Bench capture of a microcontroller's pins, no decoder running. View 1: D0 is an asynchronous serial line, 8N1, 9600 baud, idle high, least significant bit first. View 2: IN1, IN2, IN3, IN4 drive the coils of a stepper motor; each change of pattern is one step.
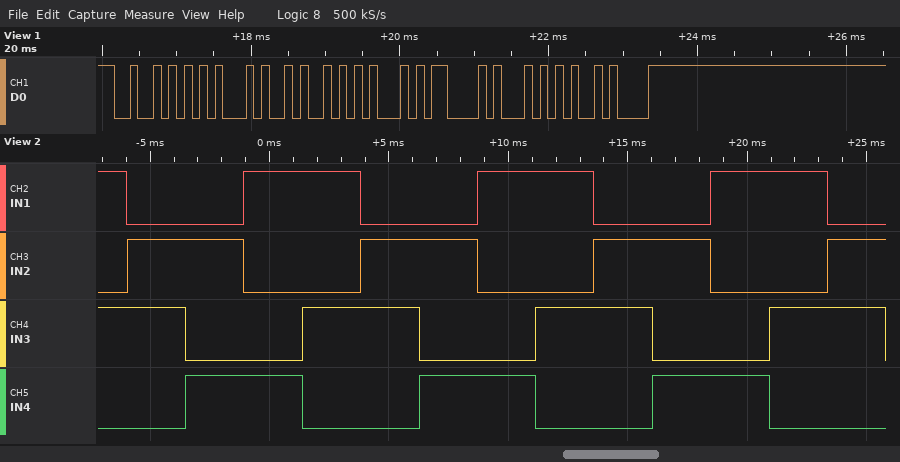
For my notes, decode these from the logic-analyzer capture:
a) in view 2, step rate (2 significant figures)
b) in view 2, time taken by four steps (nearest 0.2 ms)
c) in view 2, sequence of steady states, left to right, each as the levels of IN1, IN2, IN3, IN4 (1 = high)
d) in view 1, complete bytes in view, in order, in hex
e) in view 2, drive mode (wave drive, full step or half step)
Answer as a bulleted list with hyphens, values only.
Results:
- 410 steps/s
- 9.8 ms
- 1010 0110 0101 1001 1010 0110 0101 1001 1010 0110 0101 1001 1010 0110
- 52 45 4A 45 43 54 0A
- full step
